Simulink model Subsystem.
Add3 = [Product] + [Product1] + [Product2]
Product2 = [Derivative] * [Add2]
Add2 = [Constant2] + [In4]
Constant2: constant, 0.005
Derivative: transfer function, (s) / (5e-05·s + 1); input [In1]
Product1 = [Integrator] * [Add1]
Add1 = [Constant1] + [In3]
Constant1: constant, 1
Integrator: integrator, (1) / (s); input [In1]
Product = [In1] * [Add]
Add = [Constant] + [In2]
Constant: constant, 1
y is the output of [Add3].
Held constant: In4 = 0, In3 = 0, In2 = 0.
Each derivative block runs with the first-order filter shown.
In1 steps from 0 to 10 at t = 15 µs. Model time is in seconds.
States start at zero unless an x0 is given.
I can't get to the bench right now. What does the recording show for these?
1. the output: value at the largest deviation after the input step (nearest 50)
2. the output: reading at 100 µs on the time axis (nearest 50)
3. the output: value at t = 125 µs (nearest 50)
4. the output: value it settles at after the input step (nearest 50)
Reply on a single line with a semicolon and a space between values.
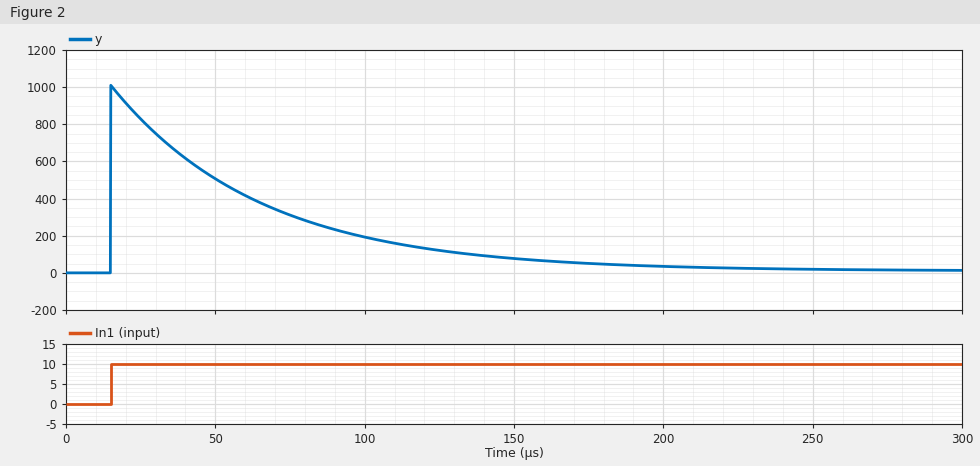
1000; 200; 100; 0
